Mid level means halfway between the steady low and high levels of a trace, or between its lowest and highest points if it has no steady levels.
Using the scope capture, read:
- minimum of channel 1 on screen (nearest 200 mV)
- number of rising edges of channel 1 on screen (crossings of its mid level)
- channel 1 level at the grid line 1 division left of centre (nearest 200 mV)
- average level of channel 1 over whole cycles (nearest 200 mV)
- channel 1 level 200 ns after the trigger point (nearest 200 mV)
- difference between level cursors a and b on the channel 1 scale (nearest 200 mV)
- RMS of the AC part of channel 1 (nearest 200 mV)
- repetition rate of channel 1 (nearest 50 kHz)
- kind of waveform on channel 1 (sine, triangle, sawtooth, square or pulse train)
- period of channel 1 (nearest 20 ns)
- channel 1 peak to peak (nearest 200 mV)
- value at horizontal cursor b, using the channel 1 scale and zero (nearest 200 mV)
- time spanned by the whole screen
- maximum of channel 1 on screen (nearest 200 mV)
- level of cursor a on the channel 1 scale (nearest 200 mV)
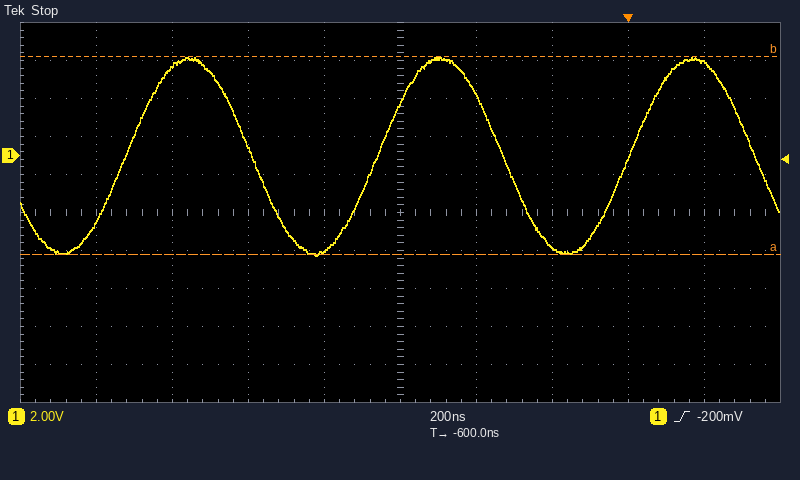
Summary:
-5.2 V
3
-5.0 V
0.0 V
4.8 V
10.4 V
3.6 V
1.50 MHz
sine
660 ns
10.4 V
5.2 V
2 µs
5.2 V
-5.2 V
